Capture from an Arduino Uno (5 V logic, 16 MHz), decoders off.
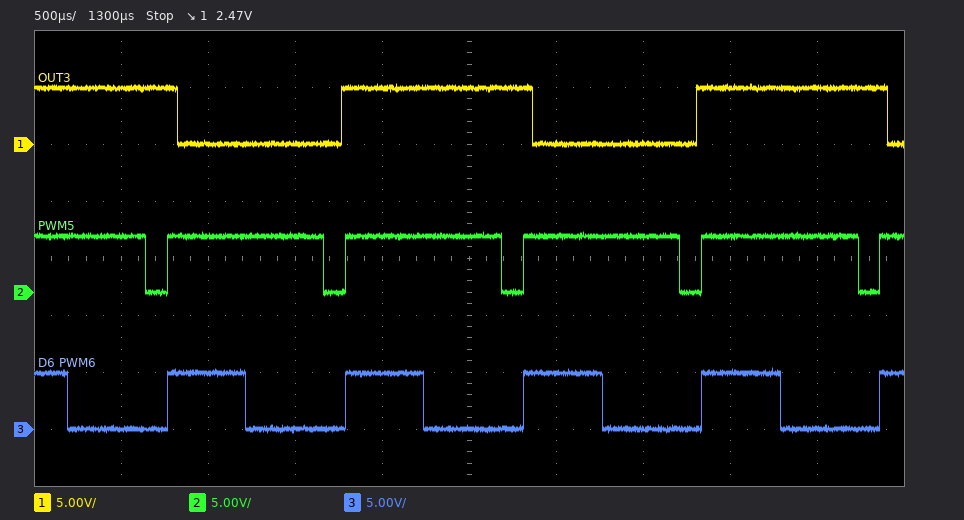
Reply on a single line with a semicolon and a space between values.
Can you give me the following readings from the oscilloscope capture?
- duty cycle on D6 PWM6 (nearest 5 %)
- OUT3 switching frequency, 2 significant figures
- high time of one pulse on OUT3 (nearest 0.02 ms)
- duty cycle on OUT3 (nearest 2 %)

45 %; 490 Hz; 1.10 ms; 54 %
